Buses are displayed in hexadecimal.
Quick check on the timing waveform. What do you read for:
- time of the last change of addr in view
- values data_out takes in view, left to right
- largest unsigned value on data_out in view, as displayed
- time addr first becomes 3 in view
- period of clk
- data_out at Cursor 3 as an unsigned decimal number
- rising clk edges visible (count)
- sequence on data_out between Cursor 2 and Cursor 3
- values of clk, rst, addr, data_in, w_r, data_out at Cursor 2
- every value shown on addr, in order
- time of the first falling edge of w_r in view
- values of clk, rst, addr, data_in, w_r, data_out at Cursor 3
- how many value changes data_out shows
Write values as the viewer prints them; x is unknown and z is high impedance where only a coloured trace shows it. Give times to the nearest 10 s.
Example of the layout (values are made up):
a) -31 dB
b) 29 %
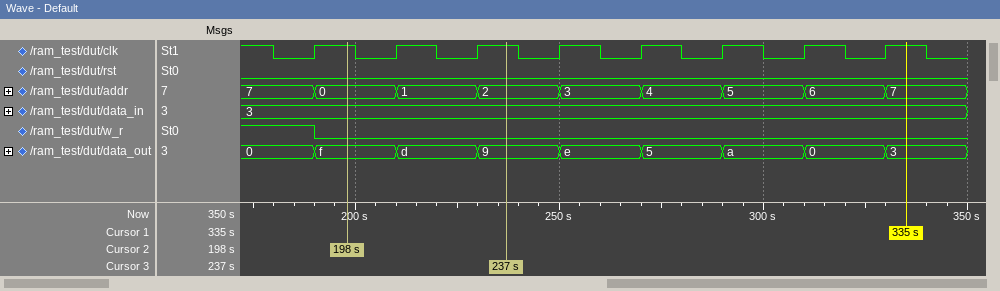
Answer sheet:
a) 330 s
b) 0, f, d, 9, e, 5, a, 0, 3
c) f
d) 250 s
e) 20 s
f) 9
g) 8
h) f, d, 9
i) clk=1, rst=0, addr=0, data_in=3, w_r=0, data_out=f
j) 7, 0, 1, 2, 3, 4, 5, 6, 7
k) 190 s
l) clk=1, rst=0, addr=2, data_in=3, w_r=0, data_out=9
m) 8
